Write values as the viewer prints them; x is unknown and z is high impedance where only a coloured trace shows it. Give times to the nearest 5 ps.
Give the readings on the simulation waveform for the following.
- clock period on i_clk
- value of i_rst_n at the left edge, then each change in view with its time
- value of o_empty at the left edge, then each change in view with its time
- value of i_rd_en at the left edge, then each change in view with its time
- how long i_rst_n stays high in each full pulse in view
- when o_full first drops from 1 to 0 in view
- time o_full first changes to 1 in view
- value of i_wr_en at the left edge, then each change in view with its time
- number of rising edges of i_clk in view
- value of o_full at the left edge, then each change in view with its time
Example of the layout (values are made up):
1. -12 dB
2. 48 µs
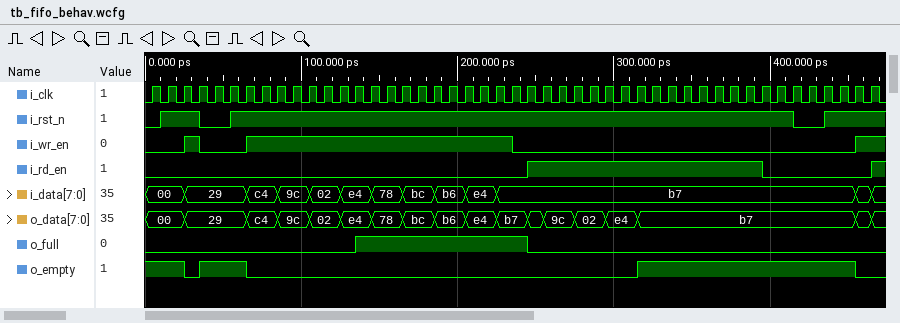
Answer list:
1. 10 ps
2. 0, 1 at 10 ps, 0 at 35 ps, 1 at 55 ps, 0 at 415 ps, 1 at 435 ps
3. 1, 0 at 25 ps, 1 at 35 ps, 0 at 65 ps, 1 at 315 ps, 0 at 455 ps
4. 0, 1 at 245 ps, 0 at 395 ps, 1 at 465 ps
5. 25 ps, 360 ps
6. 245 ps
7. 135 ps
8. 0, 1 at 25 ps, 0 at 35 ps, 1 at 65 ps, 0 at 235 ps, 1 at 455 ps
9. 47
10. 0, 1 at 135 ps, 0 at 245 ps
